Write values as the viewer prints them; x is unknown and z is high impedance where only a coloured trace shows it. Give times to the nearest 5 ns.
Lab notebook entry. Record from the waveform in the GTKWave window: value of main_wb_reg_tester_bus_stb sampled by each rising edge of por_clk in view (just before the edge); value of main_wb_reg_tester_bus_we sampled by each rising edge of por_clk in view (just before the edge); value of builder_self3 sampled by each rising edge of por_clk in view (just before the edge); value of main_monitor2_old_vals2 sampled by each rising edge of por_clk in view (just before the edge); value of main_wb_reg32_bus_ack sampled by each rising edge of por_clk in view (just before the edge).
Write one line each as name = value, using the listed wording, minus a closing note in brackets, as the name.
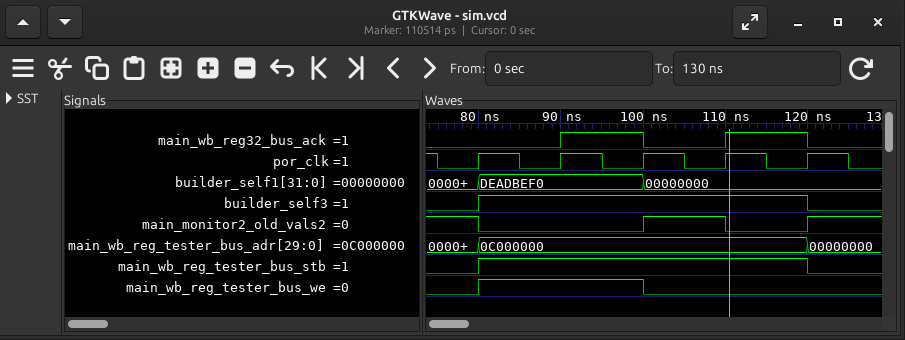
value of main_wb_reg_tester_bus_stb sampled by each rising edge of por_clk in view = 0 1 1 1 1
value of main_wb_reg_tester_bus_we sampled by each rising edge of por_clk in view = 0 1 1 0 0
value of builder_self3 sampled by each rising edge of por_clk in view = 0 1 1 1 1
value of main_monitor2_old_vals2 sampled by each rising edge of por_clk in view = 1 0 0 1 0
value of main_wb_reg32_bus_ack sampled by each rising edge of por_clk in view = 0 0 1 0 1
